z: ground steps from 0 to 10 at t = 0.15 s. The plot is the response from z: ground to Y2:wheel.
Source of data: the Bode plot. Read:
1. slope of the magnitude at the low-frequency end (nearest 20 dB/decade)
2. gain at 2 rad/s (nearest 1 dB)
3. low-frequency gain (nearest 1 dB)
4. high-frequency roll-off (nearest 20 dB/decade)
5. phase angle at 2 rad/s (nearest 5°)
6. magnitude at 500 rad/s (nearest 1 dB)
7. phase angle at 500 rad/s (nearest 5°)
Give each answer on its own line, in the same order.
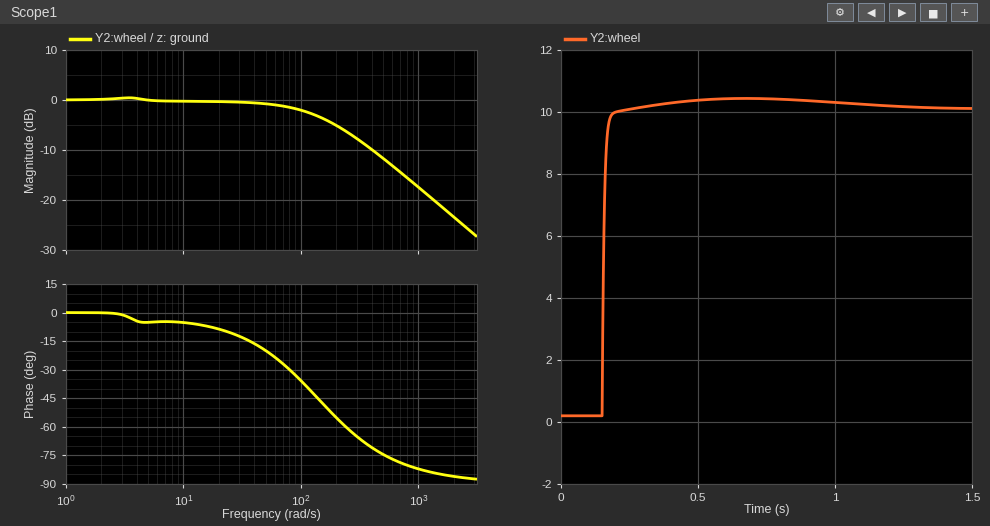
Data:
0 dB/decade
0 dB
0 dB
-20 dB/decade
0°
-12 dB
-75°
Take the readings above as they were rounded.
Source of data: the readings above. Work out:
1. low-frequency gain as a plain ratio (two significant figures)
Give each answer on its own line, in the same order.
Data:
1.0
